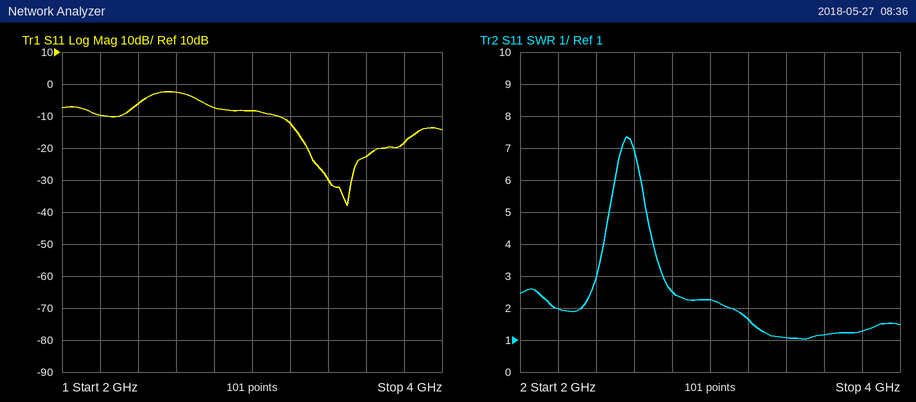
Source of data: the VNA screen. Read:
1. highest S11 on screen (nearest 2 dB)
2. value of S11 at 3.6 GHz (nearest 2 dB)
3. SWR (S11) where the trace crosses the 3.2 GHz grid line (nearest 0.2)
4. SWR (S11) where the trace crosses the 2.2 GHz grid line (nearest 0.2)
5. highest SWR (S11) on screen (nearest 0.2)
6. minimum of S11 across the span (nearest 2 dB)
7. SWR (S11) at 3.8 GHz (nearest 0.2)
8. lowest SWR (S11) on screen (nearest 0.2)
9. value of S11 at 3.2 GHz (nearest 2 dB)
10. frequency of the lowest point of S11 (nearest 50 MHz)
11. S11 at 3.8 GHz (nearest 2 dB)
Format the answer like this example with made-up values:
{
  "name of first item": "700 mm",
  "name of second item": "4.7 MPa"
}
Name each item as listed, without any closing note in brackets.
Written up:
{
  "highest S11 on screen": "-2 dB",
  "value of S11 at 3.6 GHz": "-22 dB",
  "SWR (S11) where the trace crosses the 3.2 GHz grid line": "1.6",
  "SWR (S11) where the trace crosses the 2.2 GHz grid line": "2.0",
  "highest SWR (S11) on screen": "7.4",
  "minimum of S11 across the span": "-38 dB",
  "SWR (S11) at 3.8 GHz": "1.2",
  "lowest SWR (S11) on screen": "1.0",
  "value of S11 at 3.2 GHz": "-12 dB",
  "frequency of the lowest point of S11": "3.50 GHz",
  "S11 at 3.8 GHz": "-18 dB"
}
